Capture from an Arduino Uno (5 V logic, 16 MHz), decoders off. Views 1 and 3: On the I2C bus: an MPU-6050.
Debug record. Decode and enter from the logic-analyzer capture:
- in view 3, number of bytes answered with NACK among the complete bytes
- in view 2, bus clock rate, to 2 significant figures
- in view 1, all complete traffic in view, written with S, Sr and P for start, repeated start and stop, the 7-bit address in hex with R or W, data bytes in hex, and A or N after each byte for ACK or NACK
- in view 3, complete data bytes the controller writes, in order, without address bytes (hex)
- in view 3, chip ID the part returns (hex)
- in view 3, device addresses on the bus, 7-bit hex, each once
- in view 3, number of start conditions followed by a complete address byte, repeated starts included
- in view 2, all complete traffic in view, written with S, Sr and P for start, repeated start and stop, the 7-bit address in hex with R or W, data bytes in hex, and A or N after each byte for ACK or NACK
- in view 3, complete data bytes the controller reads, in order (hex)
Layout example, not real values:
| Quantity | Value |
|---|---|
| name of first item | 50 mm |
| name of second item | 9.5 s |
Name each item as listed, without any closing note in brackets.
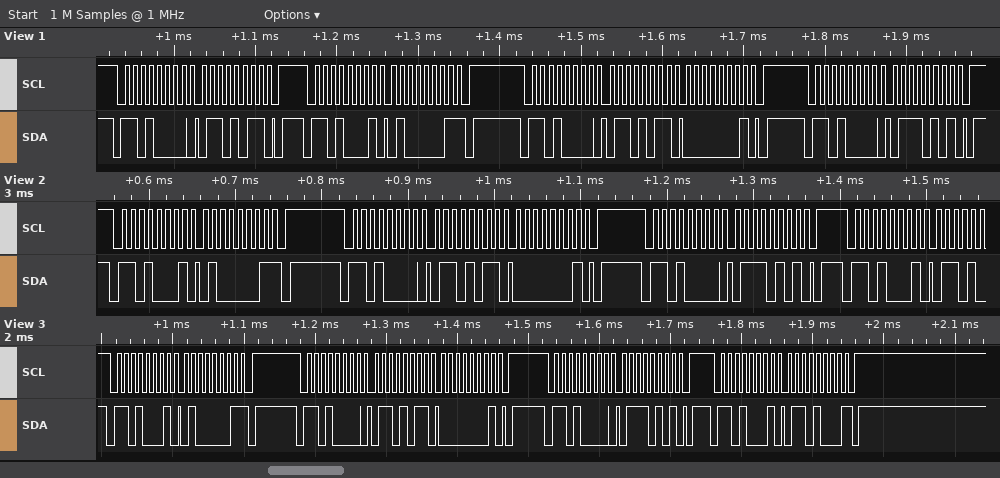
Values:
| Quantity | Value |
|---|---|
| in view 3, number of bytes answered with NACK among the complete bytes | 2 |
| in view 2, bus clock rate, to 2 significant figures | 100 kHz |
| in view 1, all complete traffic in view, written with S, Sr and P for start, repeated start and stop, the 7-bit address in hex with R or W, data bytes in hex, and A or N after each byte for ACK or NACK | S 68W A 6B A P S 68R A 41 N P S 68W A 6B A 01 A P S 68W A 75 A P |
| in view 3, complete data bytes the controller writes, in order, without address bytes | 6B 01 75 |
| in view 3, chip ID the part returns | 0x68 |
| in view 3, device addresses on the bus, 7-bit hex, each once | 0x68 |
| in view 3, number of start conditions followed by a complete address byte, repeated starts included | 4 |
| in view 2, all complete traffic in view, written with S, Sr and P for start, repeated start and stop, the 7-bit address in hex with R or W, data bytes in hex, and A or N after each byte for ACK or NACK | S 68R A 41 N P S 68W A 6B A 01 A P S 68W A 75 A P S 68R A |
| in view 3, complete data bytes the controller reads, in order | 41 68 |
